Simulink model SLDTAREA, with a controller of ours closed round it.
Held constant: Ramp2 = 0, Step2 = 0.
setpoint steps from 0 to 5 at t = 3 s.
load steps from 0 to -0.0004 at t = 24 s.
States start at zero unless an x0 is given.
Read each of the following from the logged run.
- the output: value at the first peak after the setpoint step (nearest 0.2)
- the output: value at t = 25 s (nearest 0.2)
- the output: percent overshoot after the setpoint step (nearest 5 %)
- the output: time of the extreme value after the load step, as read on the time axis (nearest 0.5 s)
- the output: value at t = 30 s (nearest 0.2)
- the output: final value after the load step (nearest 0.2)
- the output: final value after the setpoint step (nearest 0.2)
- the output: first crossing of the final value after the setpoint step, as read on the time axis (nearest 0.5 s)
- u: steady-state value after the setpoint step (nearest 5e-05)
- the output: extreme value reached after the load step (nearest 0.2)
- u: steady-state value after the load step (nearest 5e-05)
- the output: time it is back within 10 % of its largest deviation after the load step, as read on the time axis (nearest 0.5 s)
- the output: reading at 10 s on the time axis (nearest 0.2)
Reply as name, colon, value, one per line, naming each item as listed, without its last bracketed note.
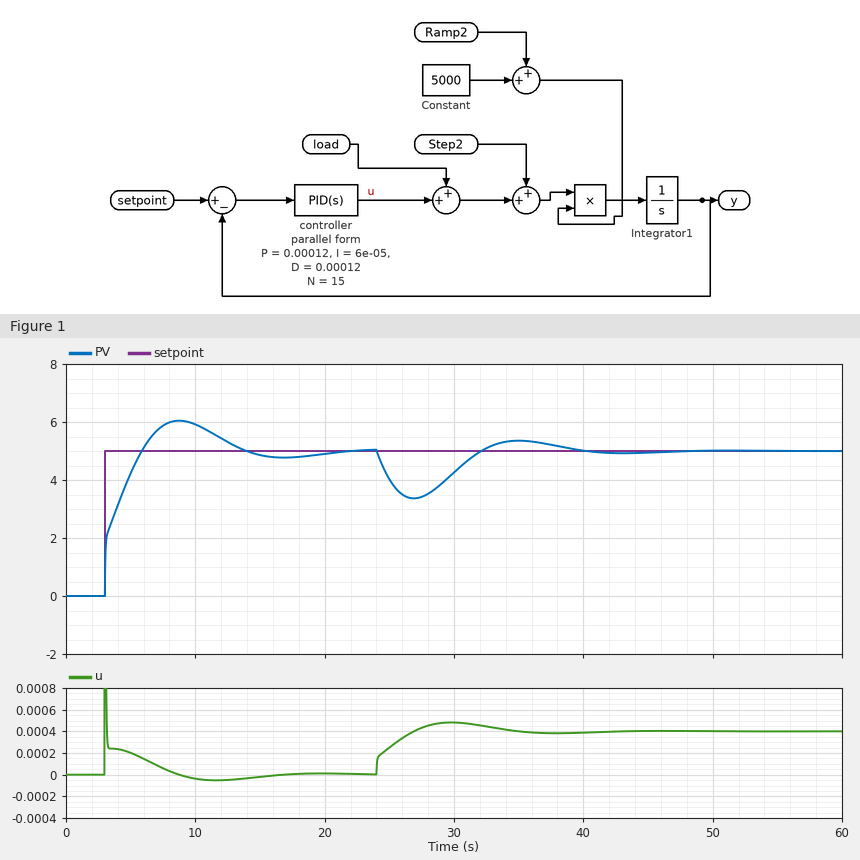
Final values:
the output: value at the first peak after the setpoint step: 6.0
the output: value at t = 25 s: 4.0
the output: percent overshoot after the setpoint step: 20 %
the output: time of the extreme value after the load step, as read on the time axis: 27.0 s
the output: value at t = 30 s: 4.2
the output: final value after the load step: 5.0
the output: final value after the setpoint step: 5.0
the output: first crossing of the final value after the setpoint step, as read on the time axis: 6.0 s
u: steady-state value after the setpoint step: 0.00000
the output: extreme value reached after the load step: 3.4
u: steady-state value after the load step: 0.00040
the output: time it is back within 10 % of its largest deviation after the load step, as read on the time axis: 38.0 s
the output: reading at 10 s on the time axis: 6.0
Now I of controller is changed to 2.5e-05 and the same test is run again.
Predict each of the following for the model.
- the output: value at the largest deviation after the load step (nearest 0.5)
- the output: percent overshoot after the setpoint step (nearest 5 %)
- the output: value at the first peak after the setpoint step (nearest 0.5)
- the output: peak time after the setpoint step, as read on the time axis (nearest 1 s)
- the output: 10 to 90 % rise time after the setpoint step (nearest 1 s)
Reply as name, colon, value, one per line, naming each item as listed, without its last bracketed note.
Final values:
the output: value at the largest deviation after the load step: 3.0
the output: percent overshoot after the setpoint step: 15 %
the output: value at the first peak after the setpoint step: 5.5
the output: peak time after the setpoint step, as read on the time axis: 11 s
the output: 10 to 90 % rise time after the setpoint step: 3 s
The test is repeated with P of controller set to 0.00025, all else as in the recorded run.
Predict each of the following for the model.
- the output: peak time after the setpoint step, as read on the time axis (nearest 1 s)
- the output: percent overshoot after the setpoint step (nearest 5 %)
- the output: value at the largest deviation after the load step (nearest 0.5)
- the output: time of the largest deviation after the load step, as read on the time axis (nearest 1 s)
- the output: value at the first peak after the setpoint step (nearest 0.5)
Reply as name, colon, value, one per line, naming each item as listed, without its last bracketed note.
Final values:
the output: peak time after the setpoint step, as read on the time axis: 8 s
the output: percent overshoot after the setpoint step: 10 %
the output: value at the largest deviation after the load step: 4.0
the output: time of the largest deviation after the load step, as read on the time axis: 26 s
the output: value at the first peak after the setpoint step: 5.5
